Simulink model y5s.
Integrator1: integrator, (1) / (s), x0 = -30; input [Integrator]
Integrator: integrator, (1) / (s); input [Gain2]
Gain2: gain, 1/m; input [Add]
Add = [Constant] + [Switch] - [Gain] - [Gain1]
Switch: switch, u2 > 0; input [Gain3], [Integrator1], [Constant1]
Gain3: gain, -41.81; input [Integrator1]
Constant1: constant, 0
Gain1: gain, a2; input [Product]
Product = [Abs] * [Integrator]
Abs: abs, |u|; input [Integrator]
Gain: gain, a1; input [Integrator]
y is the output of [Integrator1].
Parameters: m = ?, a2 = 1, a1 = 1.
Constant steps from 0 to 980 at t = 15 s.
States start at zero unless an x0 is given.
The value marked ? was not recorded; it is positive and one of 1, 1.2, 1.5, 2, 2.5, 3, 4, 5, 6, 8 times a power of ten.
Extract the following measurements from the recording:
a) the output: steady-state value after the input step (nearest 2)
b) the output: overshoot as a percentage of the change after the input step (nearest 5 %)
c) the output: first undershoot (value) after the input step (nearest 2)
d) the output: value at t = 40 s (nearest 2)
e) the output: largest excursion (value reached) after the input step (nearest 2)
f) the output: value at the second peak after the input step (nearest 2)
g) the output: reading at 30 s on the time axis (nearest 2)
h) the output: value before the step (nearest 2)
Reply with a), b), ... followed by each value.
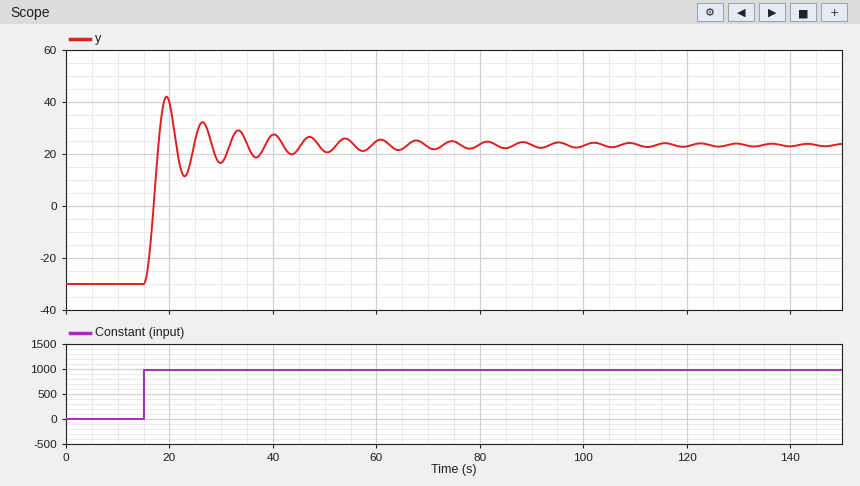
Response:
a) 24
b) 35 %
c) 12
d) 28
e) 42
f) 32
g) 16
h) -30
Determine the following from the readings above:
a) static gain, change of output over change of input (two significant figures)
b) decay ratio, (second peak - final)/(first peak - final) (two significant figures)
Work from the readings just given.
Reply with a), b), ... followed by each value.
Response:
a) 0.055
b) 0.44
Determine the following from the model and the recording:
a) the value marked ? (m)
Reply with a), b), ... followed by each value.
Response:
a) 50
